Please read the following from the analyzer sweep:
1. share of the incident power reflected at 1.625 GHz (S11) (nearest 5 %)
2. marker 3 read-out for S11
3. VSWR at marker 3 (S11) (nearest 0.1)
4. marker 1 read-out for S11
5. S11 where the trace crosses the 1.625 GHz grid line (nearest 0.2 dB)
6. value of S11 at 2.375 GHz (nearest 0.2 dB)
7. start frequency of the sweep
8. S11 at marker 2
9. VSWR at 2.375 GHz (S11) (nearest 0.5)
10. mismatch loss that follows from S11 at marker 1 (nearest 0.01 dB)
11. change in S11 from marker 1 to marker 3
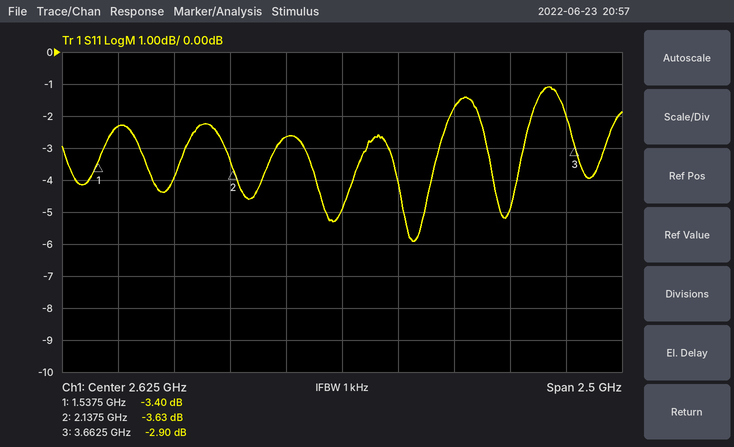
60 %
-2.90 dB
6.0
-3.40 dB
-2.4 dB
-2.6 dB
1.375 GHz
-3.63 dB
6.5
2.65 dB
0.50 dB
